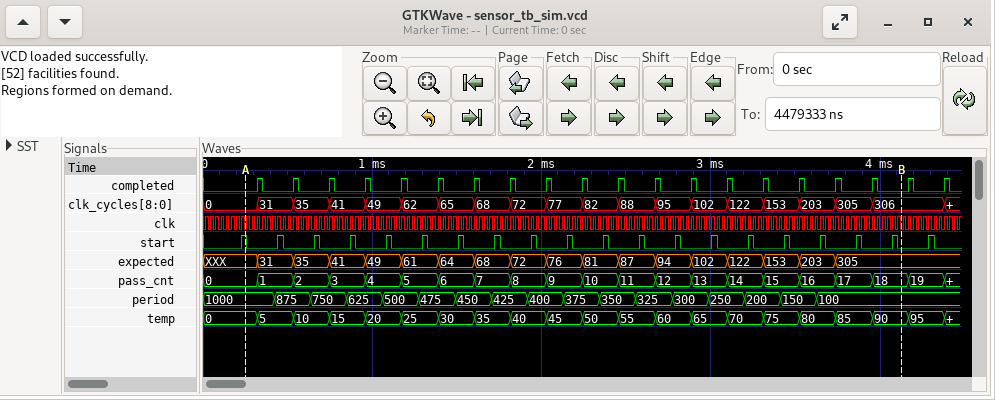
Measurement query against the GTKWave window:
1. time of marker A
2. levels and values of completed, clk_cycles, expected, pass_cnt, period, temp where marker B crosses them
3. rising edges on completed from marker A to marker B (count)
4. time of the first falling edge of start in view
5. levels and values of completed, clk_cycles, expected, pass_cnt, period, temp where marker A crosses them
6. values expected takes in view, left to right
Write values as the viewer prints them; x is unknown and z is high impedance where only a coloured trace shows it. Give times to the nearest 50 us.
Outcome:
250 us
completed=0, clk_cycles=306, expected=305, pass_cnt=18, period=100, temp=90
18
250 us
completed=0, clk_cycles=0, expected=XXX, pass_cnt=0, period=1000, temp=0
XXX, 31, 35, 41, 49, 61, 64, 68, 72, 76, 81, 87, 94, 102, 122, 153, 203, 305
